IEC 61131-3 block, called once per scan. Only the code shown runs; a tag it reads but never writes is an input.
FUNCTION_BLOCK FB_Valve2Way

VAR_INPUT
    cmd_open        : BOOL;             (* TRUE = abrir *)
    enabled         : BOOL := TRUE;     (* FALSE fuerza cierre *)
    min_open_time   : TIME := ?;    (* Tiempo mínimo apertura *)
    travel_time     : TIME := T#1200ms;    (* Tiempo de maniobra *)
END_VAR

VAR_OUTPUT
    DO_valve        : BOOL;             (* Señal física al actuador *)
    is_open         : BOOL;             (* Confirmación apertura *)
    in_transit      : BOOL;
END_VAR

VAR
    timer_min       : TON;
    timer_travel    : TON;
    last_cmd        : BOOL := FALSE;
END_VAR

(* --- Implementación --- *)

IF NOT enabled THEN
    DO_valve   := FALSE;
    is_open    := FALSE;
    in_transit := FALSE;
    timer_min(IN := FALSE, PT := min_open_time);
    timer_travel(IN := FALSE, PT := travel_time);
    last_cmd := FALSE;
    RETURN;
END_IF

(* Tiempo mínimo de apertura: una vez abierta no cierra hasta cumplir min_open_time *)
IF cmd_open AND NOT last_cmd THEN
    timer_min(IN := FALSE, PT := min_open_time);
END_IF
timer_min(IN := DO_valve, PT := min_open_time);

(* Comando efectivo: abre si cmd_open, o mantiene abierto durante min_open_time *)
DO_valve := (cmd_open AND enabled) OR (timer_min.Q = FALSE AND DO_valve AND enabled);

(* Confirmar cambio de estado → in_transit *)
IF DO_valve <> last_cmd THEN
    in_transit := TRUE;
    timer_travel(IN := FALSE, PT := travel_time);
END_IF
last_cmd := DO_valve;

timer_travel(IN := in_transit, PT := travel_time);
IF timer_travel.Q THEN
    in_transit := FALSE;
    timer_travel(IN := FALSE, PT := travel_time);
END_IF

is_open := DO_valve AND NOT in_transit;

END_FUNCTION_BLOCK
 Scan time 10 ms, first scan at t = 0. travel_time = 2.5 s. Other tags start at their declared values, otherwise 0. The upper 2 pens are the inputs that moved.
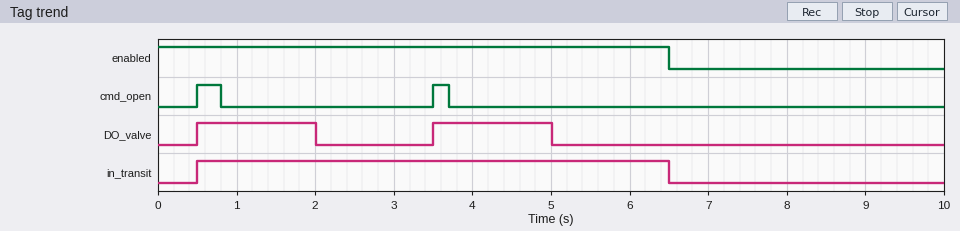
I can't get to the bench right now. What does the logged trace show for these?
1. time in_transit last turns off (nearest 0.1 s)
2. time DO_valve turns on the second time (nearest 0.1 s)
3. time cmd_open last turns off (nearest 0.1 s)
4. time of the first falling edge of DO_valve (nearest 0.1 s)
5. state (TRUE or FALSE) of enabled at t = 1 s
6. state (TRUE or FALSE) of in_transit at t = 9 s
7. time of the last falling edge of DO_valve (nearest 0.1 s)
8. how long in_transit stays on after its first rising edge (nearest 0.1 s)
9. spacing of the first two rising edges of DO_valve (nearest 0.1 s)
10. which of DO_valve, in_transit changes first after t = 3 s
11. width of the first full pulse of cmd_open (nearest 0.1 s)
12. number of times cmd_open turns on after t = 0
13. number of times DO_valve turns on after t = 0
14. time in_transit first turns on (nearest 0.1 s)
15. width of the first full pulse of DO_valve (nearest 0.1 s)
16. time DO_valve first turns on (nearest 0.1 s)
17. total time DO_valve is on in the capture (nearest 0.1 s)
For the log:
6.5 s
3.5 s
3.7 s
2.0 s
TRUE
FALSE
5.0 s
6.0 s
3.0 s
DO_valve
0.3 s
2
2
0.5 s
1.5 s
0.5 s
3.0 s
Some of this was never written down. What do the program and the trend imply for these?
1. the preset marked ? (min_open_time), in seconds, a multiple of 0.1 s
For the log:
1.5 s
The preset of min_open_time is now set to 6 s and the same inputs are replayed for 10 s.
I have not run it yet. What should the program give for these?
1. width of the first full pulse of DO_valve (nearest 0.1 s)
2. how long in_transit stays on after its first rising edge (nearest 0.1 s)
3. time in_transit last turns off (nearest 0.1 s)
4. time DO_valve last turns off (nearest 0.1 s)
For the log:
6.0 s
2.5 s
3.0 s
6.5 s
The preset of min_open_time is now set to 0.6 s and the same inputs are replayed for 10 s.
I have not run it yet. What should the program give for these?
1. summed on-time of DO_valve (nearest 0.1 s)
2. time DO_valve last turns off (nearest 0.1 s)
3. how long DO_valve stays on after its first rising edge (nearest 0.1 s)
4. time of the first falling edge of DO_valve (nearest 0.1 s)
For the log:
1.2 s
4.1 s
0.6 s
1.1 s
